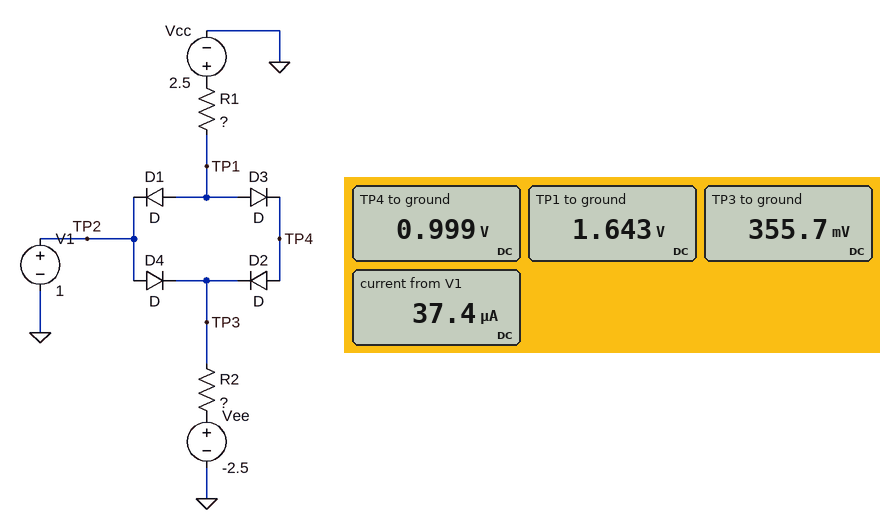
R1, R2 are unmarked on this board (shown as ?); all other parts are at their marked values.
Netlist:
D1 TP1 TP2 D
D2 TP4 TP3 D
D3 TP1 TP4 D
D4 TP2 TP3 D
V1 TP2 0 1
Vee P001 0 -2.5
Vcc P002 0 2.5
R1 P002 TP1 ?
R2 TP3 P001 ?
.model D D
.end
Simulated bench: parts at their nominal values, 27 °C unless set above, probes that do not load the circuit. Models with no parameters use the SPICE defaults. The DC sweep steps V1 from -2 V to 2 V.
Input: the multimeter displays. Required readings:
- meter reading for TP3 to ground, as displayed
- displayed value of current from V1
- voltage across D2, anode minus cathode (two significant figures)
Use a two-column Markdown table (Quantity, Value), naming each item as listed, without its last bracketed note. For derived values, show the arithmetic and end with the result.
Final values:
| Quantity | Value |
|---|---|
| meter reading for TP3 to ground, as displayed | 355.7 mV |
| displayed value of current from V1 | 37.4 µA |
| voltage across D2, anode minus cathode | 999 mV - 355.7 mV = 640 mV |
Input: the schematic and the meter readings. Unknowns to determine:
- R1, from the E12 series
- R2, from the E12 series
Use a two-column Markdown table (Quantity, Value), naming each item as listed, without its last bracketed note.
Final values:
| Quantity | Value |
|---|---|
| R1, from the E12 series | 680 Ω |
| R2, from the E12 series | 2.2 kΩ |
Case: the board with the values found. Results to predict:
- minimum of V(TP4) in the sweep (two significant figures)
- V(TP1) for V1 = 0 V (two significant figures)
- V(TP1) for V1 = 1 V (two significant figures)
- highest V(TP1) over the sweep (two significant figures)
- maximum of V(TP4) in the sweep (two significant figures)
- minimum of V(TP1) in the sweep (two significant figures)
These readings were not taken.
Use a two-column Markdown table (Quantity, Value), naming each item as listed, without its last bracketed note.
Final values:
| Quantity | Value |
|---|---|
| minimum of V(TP4) in the sweep | -1.9 V |
| V(TP1) for V1 = 0 V | 670 mV |
| V(TP1) for V1 = 1 V | 1.6 V |
| highest V(TP1) over the sweep | 2.5 V |
| maximum of V(TP4) in the sweep | 1.9 V |
| minimum of V(TP1) in the sweep | -1.3 V |
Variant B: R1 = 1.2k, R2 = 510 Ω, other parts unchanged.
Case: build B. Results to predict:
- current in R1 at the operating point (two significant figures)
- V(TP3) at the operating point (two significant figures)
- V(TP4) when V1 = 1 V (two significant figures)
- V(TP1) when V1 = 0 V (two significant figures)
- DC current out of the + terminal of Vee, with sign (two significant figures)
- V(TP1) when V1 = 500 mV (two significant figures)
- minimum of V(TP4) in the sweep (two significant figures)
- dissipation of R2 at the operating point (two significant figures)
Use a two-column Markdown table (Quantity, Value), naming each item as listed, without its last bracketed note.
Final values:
| Quantity | Value |
|---|---|
| current in R1 at the operating point | 760 µA |
| V(TP3) at the operating point | 300 mV |
| V(TP4) when V1 = 1 V | 950 mV |
| V(TP1) when V1 = 0 V | 640 mV |
| DC current out of the + terminal of Vee, with sign | -5.5 mA |
| V(TP1) when V1 = 500 mV | 1.1 V |
| minimum of V(TP4) in the sweep | -1.9 V |
| dissipation of R2 at the operating point | 15 mW |
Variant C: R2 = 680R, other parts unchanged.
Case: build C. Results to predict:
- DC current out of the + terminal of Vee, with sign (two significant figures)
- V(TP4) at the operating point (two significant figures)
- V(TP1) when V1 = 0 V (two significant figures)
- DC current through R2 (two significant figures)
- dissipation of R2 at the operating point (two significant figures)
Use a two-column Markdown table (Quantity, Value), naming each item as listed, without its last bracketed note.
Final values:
| Quantity | Value |
|---|---|
| DC current out of the + terminal of Vee, with sign | -4.1 mA |
| V(TP4) at the operating point | 970 mV |
| V(TP1) when V1 = 0 V | 660 mV |
| DC current through R2 | 4.1 mA |
| dissipation of R2 at the operating point | 12 mW |
